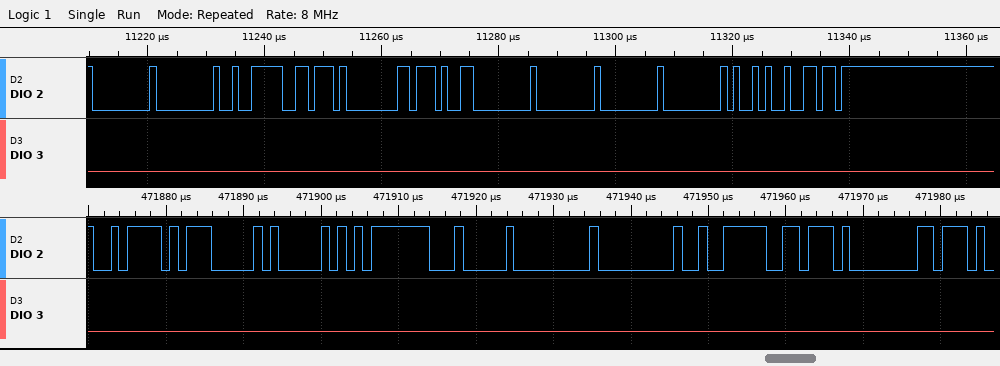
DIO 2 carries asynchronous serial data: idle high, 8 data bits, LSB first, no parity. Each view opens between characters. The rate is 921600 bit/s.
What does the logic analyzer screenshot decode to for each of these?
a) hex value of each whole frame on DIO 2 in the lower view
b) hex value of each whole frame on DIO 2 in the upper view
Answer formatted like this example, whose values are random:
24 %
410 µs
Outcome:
7A, 07, 41, FD, 04, 00, 00, F2, 76, 80
00, 00, F2, 76, 80, 97, 00, 00, 00, 00, 29, B6
